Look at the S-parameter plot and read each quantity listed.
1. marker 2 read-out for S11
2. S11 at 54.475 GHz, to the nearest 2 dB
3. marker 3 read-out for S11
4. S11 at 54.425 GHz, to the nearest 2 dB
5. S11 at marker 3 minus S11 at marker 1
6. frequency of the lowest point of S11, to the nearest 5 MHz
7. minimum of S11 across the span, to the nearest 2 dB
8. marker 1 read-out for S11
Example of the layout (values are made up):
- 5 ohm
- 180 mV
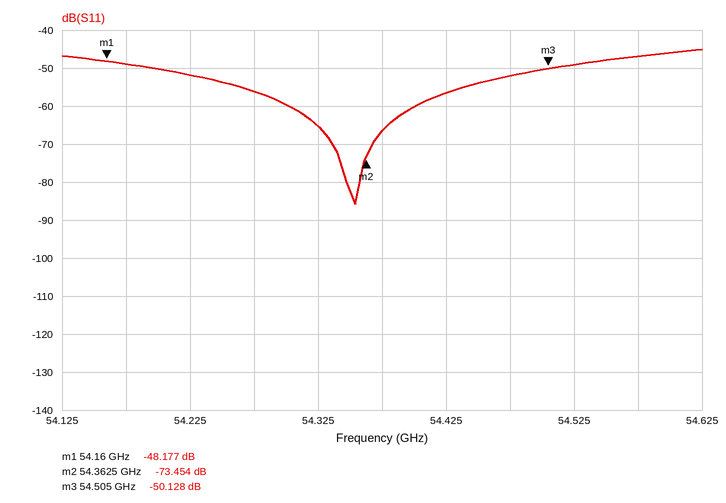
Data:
- -73.454 dB
- -52 dB
- -50.128 dB
- -56 dB
- -1.951 dB
- 54.355 GHz
- -86 dB
- -48.177 dB
